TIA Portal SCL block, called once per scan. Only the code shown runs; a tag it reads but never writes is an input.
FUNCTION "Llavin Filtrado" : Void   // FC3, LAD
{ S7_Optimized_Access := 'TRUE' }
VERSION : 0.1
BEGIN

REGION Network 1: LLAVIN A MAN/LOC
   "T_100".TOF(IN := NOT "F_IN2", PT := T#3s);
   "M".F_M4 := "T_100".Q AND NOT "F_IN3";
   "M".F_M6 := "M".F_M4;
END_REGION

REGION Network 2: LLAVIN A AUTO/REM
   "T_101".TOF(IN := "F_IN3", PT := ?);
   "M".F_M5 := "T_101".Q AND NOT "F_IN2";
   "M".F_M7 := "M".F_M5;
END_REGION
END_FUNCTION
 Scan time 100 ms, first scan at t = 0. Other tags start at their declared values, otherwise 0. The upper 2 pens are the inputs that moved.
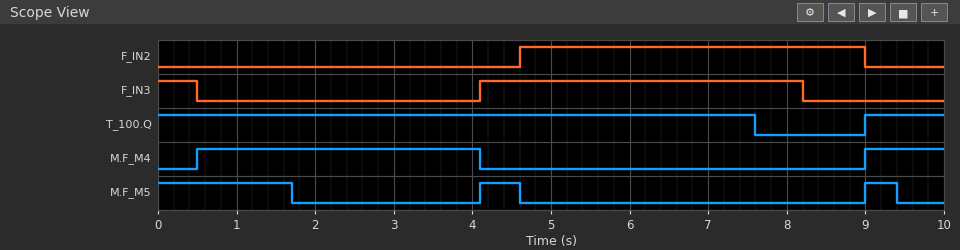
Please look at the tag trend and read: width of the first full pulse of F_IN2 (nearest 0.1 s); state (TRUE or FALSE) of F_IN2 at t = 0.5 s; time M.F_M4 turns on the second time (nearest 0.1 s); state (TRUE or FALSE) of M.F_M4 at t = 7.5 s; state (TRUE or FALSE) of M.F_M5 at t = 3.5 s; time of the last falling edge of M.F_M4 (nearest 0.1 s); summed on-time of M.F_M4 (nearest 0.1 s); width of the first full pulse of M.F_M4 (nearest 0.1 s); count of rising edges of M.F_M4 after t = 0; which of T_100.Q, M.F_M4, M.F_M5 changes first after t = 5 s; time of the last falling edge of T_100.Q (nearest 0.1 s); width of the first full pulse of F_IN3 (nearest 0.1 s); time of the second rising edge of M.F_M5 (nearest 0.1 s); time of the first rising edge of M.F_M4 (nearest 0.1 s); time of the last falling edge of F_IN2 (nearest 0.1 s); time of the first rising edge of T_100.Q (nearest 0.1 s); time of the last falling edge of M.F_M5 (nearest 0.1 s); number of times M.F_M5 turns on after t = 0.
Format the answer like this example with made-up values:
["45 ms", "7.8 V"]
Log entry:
["4.4 s", "FALSE", "9.0 s", "FALSE", "FALSE", "4.1 s", "4.6 s", "3.6 s", "2", "T_100.Q", "7.6 s", "4.1 s", "9.0 s", "0.5 s", "9.0 s", "9.0 s", "9.4 s", "2"]
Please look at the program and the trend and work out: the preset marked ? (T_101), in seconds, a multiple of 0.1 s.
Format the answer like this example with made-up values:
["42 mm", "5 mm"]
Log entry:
["1.2 s"]
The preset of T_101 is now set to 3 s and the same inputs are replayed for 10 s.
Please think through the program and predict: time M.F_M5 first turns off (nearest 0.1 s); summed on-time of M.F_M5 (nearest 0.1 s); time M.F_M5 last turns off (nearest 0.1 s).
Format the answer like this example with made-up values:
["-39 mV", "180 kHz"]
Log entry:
["3.5 s", "5.0 s", "4.6 s"]
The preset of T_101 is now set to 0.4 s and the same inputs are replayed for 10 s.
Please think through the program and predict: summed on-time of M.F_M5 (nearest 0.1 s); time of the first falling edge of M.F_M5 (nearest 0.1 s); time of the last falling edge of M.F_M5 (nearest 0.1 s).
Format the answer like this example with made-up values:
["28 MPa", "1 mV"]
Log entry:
["1.4 s", "0.9 s", "4.6 s"]
